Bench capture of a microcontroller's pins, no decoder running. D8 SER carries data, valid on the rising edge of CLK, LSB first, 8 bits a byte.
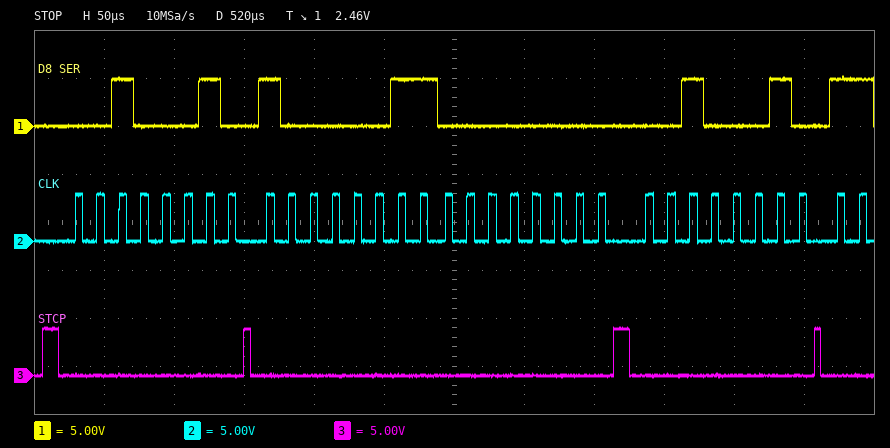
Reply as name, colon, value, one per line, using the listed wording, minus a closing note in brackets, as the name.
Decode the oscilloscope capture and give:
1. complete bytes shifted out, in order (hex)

complete bytes shifted out, in order: 44 C1 00 44
